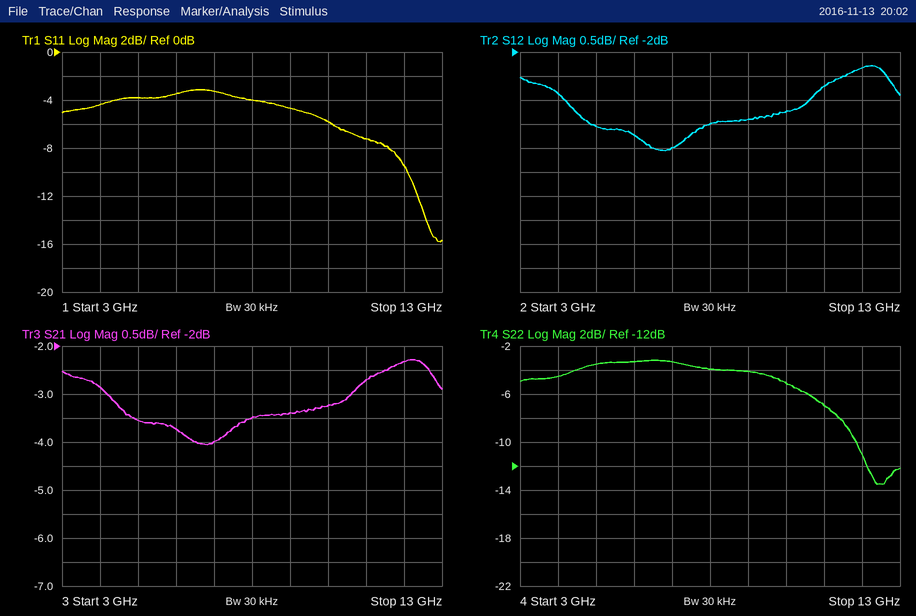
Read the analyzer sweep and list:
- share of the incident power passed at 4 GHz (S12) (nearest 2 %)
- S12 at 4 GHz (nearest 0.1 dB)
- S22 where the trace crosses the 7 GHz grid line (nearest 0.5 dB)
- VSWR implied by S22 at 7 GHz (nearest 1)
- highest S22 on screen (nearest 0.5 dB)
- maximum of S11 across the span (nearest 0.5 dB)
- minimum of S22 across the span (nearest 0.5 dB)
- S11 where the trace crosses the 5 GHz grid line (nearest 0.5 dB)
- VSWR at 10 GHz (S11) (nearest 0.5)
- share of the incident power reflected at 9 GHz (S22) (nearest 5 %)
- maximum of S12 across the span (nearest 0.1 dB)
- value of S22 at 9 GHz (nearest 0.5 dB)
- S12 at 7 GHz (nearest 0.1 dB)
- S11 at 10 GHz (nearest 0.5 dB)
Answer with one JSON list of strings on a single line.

["52 %", "-2.9 dB", "-3.5 dB", "5", "-3.0 dB", "-3.0 dB", "-13.5 dB", "-4.0 dB", "3.0", "40 %", "-2.3 dB", "-4.0 dB", "-4.0 dB", "-6.0 dB"]
